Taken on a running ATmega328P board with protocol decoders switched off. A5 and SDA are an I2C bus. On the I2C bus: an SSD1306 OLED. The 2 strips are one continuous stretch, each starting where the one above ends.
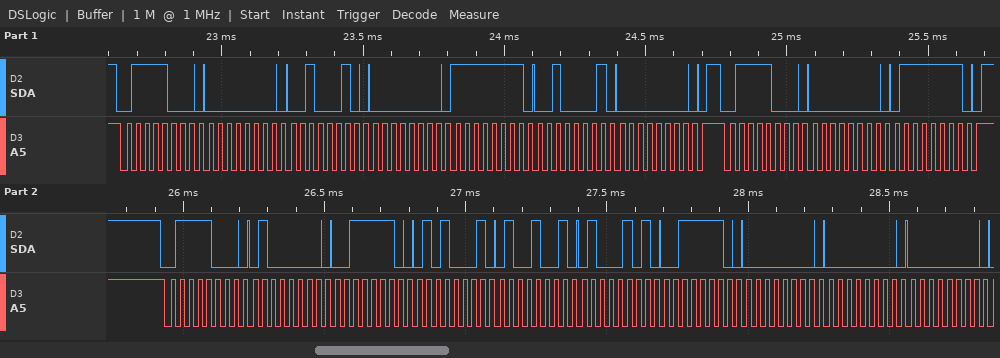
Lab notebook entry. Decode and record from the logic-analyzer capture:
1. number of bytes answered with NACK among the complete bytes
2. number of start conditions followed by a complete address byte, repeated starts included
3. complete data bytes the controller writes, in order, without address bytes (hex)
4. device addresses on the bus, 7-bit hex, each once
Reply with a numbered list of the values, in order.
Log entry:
1. 0
2. 3
3. 00 22 00 FF 21 00 00 7F 40 3E 51 49 45 3E 00 00 00
4. 0x3C
